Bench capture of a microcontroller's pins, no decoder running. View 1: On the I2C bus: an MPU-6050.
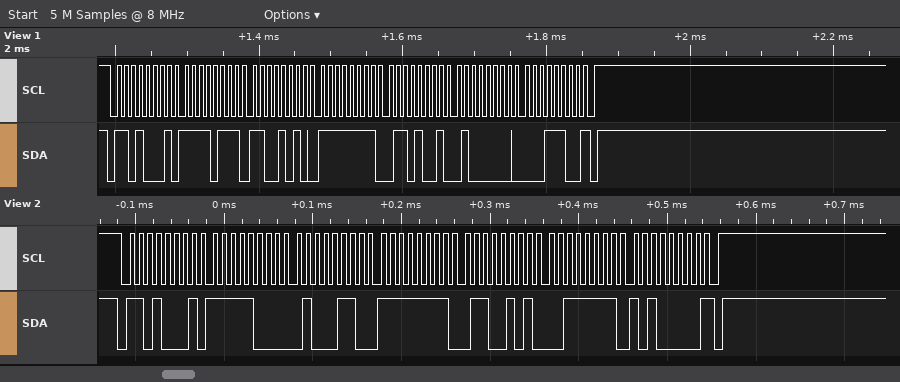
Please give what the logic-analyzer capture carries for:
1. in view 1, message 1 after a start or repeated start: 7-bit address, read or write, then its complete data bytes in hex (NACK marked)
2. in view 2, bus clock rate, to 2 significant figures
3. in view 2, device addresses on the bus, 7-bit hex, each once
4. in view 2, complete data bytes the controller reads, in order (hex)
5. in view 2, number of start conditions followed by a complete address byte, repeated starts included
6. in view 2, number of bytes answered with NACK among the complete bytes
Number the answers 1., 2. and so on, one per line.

1. 0x68 read: F7 CA FF 69 40 1C NACK
2. 100 kHz
3. 0x68
4. F8 46 FF 65 3F A0
5. 1
6. 1
